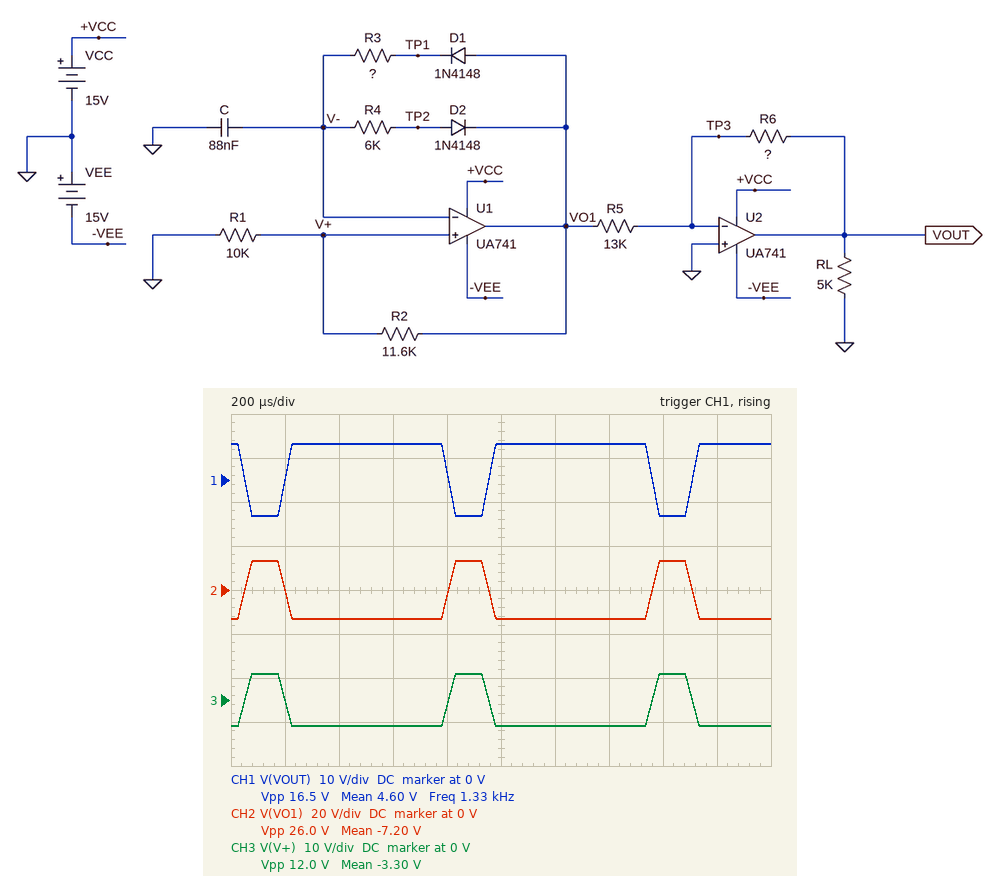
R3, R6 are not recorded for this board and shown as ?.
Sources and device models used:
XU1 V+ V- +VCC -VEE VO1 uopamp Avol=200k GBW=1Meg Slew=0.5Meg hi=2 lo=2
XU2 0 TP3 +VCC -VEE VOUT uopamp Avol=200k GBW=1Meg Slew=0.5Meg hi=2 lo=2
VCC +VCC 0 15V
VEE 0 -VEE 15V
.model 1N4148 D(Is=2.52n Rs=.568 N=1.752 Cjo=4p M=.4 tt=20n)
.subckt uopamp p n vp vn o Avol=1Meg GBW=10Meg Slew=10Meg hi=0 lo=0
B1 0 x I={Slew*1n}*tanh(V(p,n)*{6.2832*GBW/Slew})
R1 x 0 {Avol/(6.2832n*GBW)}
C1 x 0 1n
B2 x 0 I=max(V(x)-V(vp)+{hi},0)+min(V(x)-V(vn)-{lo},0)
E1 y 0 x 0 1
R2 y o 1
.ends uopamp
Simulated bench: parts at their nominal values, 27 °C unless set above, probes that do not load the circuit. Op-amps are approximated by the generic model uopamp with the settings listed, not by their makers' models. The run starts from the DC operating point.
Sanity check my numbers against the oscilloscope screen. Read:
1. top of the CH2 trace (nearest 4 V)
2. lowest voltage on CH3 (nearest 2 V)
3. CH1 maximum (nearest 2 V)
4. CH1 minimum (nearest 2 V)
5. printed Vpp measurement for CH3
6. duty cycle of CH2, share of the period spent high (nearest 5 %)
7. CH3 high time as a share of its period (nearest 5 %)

12 V
-6 V
8 V
-8 V
12.0 V
20 %
20 %
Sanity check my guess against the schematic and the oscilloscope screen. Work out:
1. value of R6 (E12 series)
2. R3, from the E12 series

8.2 kΩ
1.2 kΩ
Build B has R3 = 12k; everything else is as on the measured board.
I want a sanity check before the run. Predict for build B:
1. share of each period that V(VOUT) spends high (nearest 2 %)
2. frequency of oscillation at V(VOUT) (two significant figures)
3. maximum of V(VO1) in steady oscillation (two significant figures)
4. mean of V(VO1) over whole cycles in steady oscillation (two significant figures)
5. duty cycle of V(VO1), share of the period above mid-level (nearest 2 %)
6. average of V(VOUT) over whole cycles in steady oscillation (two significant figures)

34 %
570 Hz
13 V
4.2 V
66 %
-2.6 V
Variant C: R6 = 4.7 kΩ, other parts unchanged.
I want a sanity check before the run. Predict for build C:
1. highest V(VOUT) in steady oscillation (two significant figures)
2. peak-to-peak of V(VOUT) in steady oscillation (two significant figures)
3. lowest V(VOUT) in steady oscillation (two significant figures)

4.7 V
9.4 V
-4.7 V
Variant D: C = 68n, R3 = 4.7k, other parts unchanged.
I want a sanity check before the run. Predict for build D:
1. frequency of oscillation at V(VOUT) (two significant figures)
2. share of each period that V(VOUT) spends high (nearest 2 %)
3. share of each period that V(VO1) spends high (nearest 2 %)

1.2 kHz
56 %
44 %
